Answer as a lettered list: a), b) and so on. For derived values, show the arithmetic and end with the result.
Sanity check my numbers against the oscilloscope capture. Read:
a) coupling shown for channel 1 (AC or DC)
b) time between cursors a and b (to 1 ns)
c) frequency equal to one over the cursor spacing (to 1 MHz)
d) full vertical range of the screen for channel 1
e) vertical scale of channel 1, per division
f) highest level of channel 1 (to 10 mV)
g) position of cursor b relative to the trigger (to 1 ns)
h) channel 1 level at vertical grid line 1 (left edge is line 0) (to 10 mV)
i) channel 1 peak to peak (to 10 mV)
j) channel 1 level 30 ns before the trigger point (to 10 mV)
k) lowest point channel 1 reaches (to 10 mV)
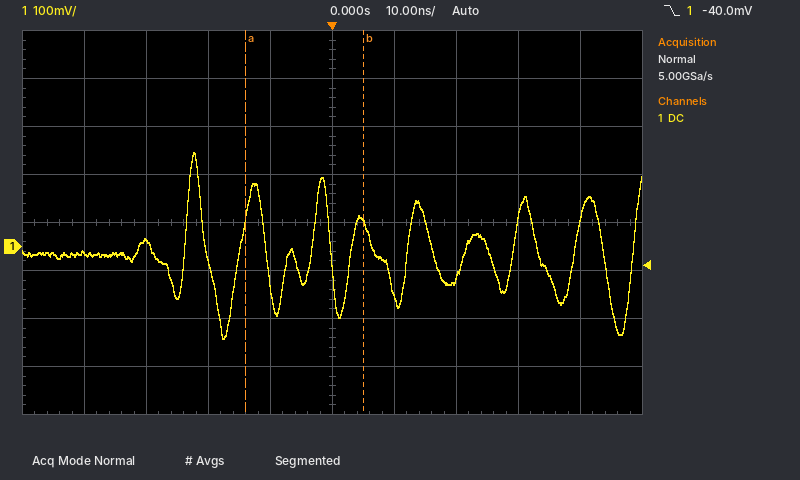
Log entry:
a) DC
b) 19 ns
c) 1 / 19 ns ≈ 53 MHz
d) 800 mV
e) 100 mV
f) 200 mV
g) +5 ns
h) -10 mV
i) 200 mV − (-190 mV) = 390 mV
j) 10 mV
k) -190 mV
